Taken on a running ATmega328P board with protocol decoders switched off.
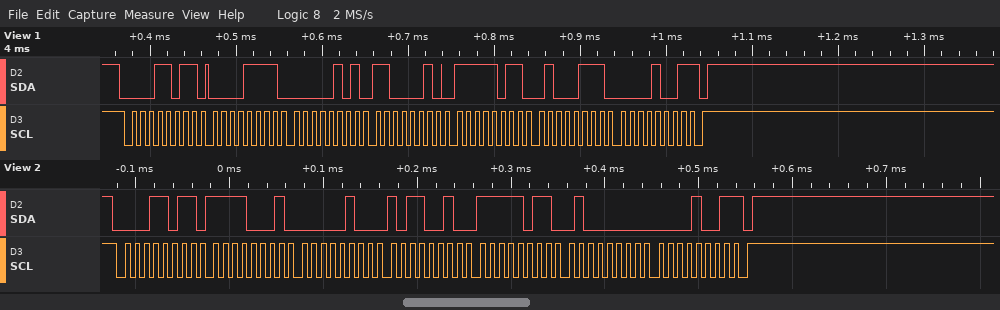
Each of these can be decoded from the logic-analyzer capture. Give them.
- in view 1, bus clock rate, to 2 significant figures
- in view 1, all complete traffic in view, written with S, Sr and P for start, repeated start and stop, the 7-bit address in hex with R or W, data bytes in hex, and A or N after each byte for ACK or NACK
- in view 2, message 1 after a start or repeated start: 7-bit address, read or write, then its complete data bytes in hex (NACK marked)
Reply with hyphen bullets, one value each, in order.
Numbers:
- 100 kHz
- S 0DR A 0F A 05 A C2 A FB A 47 A 09 N P
- 0x0D read: F1 04 B2 FB 40 09 NACK
